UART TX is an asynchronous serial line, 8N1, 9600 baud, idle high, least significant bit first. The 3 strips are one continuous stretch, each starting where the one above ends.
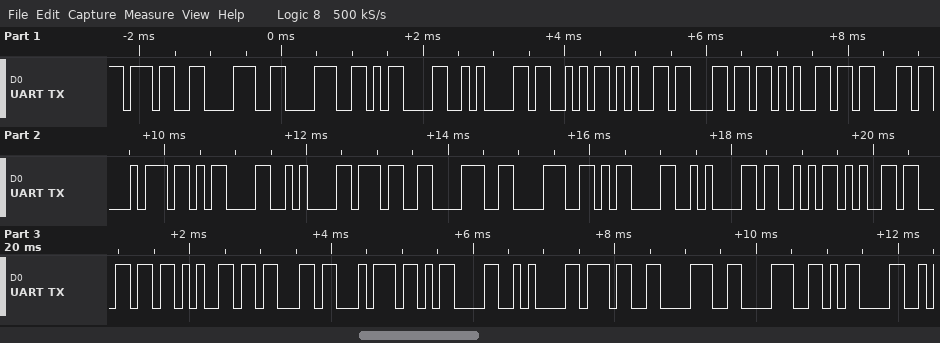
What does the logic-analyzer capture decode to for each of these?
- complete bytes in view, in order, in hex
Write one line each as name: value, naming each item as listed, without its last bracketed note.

complete bytes in view, in order, in hex: 37 38 38 0D 0A 53 65 6C 65 63 74 0D 0A 37 38 38 0D 0A 53 65 6C 65 63 74 0D 0A 37 38 38 0D
